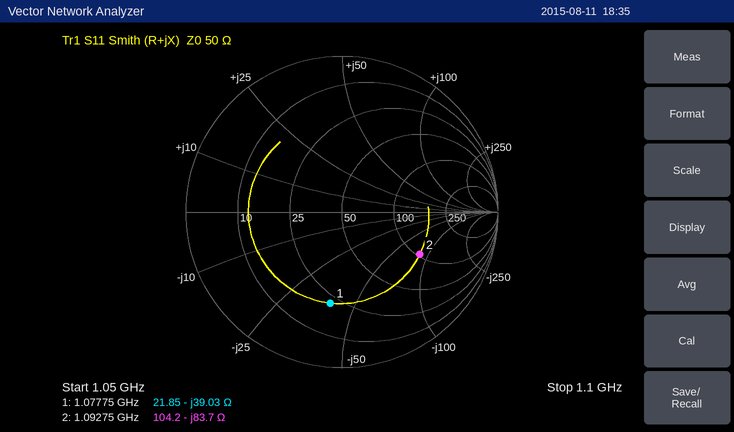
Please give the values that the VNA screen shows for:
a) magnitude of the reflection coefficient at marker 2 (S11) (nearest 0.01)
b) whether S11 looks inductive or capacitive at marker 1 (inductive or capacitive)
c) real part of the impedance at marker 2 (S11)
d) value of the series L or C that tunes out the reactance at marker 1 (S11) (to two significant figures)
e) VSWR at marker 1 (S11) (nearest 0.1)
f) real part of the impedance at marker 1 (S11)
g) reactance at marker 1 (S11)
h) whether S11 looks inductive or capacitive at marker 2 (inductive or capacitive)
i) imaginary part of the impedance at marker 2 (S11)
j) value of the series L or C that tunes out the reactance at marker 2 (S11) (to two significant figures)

0.57
capacitive
104.2 Ω
5.8 nH
3.9
21.85 Ω
-39.03 Ω
capacitive
-83.7 Ω
12 nH
